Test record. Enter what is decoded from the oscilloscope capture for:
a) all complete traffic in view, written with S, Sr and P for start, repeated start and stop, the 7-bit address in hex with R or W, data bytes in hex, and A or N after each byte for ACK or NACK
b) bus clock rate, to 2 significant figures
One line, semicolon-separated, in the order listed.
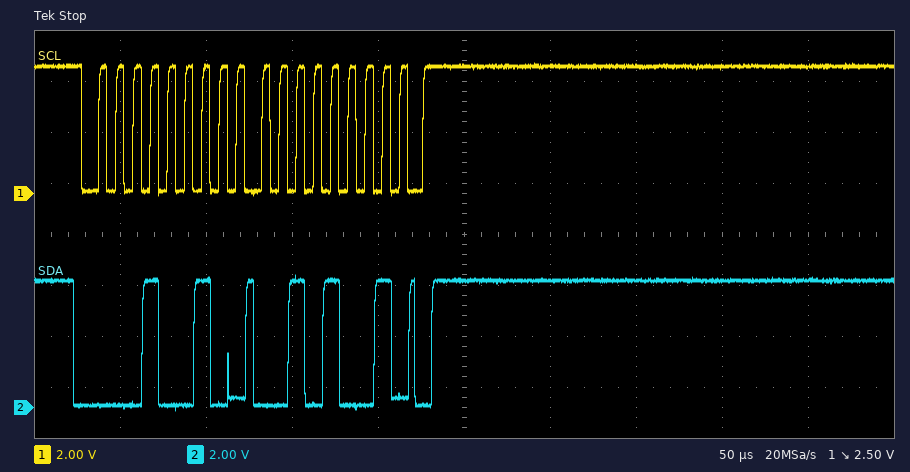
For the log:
S 09W A 29 A P; 100 kHz
